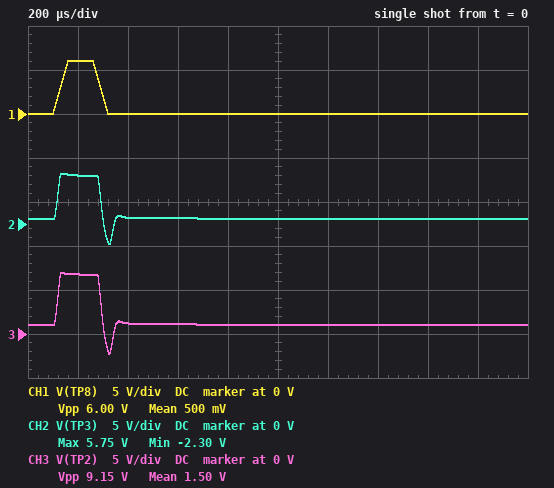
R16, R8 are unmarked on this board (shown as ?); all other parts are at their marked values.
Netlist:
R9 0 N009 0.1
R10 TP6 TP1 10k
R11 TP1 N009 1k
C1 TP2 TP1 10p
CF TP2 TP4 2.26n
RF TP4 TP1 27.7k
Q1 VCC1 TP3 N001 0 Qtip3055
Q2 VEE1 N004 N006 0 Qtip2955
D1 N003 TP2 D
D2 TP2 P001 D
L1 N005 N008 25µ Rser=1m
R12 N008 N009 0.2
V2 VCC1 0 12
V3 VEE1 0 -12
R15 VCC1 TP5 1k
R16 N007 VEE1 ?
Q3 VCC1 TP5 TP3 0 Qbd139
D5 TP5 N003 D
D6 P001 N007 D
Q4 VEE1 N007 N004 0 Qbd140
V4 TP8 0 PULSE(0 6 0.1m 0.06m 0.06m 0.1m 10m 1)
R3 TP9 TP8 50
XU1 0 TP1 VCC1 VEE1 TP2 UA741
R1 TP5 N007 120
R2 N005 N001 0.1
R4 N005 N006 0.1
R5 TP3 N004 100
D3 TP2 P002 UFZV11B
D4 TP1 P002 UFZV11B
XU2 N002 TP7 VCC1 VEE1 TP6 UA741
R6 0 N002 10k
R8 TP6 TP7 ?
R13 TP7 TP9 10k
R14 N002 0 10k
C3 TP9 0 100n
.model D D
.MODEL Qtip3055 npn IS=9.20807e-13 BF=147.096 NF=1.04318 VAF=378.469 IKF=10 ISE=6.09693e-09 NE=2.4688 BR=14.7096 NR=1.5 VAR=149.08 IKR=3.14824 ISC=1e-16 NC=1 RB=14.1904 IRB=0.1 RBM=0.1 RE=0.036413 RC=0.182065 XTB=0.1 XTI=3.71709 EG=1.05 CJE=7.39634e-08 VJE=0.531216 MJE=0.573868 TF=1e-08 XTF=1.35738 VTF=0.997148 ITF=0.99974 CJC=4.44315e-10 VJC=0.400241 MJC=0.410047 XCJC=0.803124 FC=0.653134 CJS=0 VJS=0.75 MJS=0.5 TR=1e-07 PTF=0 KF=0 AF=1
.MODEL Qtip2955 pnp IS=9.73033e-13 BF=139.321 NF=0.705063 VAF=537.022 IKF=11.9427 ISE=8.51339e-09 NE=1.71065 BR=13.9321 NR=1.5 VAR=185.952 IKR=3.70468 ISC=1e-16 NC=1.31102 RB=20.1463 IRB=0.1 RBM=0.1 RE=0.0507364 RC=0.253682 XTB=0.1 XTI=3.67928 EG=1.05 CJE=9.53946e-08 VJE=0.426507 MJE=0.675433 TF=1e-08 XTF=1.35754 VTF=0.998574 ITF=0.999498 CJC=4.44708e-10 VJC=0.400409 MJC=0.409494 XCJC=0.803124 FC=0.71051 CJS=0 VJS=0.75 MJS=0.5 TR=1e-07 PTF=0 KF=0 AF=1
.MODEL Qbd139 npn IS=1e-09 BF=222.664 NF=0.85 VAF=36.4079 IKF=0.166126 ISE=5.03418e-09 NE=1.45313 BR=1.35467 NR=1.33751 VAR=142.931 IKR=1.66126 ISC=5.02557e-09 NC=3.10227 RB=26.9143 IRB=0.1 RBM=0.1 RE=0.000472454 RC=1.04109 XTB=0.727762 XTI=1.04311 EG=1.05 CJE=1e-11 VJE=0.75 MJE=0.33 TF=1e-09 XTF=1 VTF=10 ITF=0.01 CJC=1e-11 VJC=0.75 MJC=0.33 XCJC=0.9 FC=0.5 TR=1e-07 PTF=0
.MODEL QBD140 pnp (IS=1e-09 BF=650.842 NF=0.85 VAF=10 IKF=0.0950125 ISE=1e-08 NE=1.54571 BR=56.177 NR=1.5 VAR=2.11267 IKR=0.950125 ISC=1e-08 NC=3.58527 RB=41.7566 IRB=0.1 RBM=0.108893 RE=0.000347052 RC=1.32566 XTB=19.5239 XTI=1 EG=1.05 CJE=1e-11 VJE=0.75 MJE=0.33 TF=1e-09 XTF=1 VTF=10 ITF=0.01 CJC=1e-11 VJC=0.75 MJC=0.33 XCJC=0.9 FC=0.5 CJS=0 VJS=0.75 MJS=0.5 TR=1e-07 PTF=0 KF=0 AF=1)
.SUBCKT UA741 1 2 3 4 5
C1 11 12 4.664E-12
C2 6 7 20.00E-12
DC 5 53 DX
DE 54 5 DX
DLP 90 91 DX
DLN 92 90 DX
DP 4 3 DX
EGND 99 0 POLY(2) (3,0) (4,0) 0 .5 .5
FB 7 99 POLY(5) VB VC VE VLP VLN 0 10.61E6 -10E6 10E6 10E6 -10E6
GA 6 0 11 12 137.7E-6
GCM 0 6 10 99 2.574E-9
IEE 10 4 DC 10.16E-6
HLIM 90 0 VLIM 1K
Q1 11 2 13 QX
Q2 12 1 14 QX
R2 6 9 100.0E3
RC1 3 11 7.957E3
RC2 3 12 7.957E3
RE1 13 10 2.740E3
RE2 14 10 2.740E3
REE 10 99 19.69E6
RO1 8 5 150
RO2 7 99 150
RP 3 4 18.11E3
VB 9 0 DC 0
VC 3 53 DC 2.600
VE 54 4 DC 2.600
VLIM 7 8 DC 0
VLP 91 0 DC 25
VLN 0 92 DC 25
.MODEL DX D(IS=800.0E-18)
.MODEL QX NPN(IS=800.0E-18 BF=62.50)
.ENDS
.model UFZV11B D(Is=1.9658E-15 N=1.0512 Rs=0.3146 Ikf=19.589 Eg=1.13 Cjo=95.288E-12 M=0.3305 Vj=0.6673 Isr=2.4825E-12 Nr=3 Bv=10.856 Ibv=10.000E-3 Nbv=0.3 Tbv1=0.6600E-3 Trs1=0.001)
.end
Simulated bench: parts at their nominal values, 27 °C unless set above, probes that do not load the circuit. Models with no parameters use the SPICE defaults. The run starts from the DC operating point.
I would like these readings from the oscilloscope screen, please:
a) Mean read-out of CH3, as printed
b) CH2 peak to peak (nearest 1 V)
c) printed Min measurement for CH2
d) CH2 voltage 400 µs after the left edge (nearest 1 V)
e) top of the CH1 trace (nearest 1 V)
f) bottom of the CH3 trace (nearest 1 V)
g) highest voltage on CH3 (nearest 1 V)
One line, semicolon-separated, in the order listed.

1.50 V; 8 V; -2.30 V; 1 V; 6 V; -2 V; 7 V
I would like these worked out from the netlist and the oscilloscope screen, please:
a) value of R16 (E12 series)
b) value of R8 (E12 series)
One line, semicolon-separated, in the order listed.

560 Ω; 18 kΩ
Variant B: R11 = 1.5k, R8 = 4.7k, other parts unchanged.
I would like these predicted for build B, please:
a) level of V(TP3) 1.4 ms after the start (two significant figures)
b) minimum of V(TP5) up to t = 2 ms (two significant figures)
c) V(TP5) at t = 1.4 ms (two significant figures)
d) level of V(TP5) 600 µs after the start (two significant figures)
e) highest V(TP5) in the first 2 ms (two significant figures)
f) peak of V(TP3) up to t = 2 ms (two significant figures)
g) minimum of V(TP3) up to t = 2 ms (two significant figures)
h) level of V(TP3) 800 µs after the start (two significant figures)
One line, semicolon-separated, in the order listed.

590 mV; 210 mV; 930 mV; 990 mV; 4.3 V; 3.9 V; -150 mV; 620 mV
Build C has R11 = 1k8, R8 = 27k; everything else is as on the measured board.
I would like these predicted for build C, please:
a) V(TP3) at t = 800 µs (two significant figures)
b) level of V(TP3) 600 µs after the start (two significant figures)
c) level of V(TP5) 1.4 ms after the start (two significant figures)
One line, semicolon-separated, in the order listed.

630 mV; 680 mV; 930 mV
